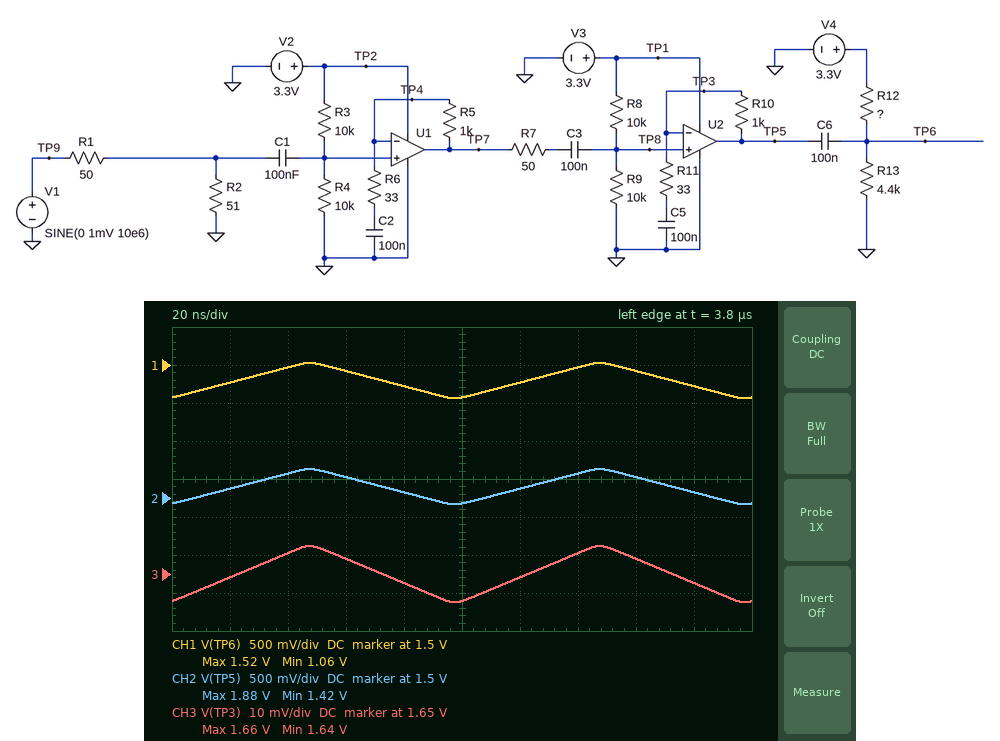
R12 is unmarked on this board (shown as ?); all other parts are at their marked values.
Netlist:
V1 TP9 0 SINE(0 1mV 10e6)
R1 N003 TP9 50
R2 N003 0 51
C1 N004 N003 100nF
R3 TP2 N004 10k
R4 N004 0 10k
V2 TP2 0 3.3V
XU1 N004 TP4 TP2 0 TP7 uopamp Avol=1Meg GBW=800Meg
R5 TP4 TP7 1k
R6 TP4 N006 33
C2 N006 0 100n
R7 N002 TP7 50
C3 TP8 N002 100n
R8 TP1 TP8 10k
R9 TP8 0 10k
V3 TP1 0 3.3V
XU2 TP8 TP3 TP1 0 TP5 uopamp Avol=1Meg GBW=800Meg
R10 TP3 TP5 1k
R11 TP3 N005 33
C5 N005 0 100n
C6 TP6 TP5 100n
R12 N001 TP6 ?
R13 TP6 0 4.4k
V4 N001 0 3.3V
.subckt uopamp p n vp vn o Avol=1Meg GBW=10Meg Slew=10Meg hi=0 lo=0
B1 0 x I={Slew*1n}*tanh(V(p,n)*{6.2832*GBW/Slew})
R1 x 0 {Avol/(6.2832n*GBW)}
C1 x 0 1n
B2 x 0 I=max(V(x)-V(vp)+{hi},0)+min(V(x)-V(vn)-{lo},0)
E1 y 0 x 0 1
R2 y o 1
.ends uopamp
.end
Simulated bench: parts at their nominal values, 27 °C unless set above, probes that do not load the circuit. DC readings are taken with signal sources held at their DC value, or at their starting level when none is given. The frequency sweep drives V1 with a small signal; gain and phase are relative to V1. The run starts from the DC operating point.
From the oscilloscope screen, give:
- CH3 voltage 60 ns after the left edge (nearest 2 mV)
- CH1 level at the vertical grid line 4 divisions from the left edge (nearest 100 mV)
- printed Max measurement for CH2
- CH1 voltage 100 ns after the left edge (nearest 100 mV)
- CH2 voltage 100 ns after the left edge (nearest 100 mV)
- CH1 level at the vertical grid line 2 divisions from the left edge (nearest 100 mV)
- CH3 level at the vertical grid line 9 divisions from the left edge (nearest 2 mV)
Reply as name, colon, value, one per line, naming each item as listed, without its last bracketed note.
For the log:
CH3 voltage 60 ns after the left edge: 1.654 V
CH1 level at the vertical grid line 4 divisions from the left edge: 1.2 V
printed Max measurement for CH2: 1.88 V
CH1 voltage 100 ns after the left edge: 1.1 V
CH2 voltage 100 ns after the left edge: 1.4 V
CH1 level at the vertical grid line 2 divisions from the left edge: 1.5 V
CH3 level at the vertical grid line 9 divisions from the left edge: 1.648 V
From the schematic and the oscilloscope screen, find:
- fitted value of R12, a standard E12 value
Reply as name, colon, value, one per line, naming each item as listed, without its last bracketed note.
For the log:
fitted value of R12, a standard E12 value: 6.8 kΩ
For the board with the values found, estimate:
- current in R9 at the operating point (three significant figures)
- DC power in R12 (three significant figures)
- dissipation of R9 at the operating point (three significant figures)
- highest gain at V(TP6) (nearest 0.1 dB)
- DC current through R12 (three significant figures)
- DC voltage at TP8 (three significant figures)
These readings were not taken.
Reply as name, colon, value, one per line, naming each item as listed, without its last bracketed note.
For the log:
current in R9 at the operating point: 165 µA
DC power in R12: 590 µW
dissipation of R9 at the operating point: 272 µW
highest gain at V(TP6): 53.8 dB
DC current through R12: 295 µA
DC voltage at TP8: 1.65 V
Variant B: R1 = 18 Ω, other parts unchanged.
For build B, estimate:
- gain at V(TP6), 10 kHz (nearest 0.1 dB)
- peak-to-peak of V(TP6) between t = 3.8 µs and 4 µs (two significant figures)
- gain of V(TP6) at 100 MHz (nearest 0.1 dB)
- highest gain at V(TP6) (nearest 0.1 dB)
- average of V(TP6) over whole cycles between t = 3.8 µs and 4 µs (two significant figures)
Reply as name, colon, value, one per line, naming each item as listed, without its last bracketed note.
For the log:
gain at V(TP6), 10 kHz: 29.6 dB
peak-to-peak of V(TP6) between t = 3.8 µs and 4 µs: 480 mV
gain of V(TP6) at 100 MHz: 32.8 dB
highest gain at V(TP6): 57.1 dB
average of V(TP6) over whole cycles between t = 3.8 µs and 4 µs: 1.3 V
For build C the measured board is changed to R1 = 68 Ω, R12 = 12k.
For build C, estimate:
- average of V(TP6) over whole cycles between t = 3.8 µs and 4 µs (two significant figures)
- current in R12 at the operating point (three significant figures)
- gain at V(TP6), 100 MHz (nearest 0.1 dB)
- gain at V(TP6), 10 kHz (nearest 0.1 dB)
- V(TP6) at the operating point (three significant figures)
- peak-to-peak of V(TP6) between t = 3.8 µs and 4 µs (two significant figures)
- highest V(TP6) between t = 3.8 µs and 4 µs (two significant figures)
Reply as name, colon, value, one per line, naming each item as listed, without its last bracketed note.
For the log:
average of V(TP6) over whole cycles between t = 3.8 µs and 4 µs: 880 mV
current in R12 at the operating point: 201 µA
gain at V(TP6), 100 MHz: 28.1 dB
gain at V(TP6), 10 kHz: 24.8 dB
V(TP6) at the operating point: 885 mV
peak-to-peak of V(TP6) between t = 3.8 µs and 4 µs: 450 mV
highest V(TP6) between t = 3.8 µs and 4 µs: 1.1 V
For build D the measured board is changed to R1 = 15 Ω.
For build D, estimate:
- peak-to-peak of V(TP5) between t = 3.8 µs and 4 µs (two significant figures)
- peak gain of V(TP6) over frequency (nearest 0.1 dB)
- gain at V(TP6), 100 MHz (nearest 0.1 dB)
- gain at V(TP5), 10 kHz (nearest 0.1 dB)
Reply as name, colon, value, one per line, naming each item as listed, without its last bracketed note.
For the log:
peak-to-peak of V(TP5) between t = 3.8 µs and 4 µs: 480 mV
peak gain of V(TP6) over frequency: 57.5 dB
gain at V(TP6), 100 MHz: 33.2 dB
gain at V(TP5), 10 kHz: 30.0 dB
